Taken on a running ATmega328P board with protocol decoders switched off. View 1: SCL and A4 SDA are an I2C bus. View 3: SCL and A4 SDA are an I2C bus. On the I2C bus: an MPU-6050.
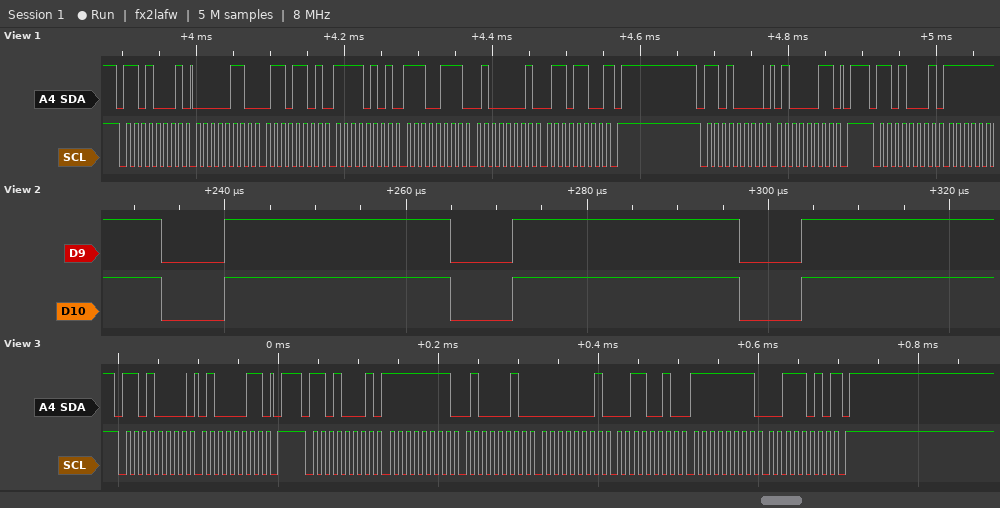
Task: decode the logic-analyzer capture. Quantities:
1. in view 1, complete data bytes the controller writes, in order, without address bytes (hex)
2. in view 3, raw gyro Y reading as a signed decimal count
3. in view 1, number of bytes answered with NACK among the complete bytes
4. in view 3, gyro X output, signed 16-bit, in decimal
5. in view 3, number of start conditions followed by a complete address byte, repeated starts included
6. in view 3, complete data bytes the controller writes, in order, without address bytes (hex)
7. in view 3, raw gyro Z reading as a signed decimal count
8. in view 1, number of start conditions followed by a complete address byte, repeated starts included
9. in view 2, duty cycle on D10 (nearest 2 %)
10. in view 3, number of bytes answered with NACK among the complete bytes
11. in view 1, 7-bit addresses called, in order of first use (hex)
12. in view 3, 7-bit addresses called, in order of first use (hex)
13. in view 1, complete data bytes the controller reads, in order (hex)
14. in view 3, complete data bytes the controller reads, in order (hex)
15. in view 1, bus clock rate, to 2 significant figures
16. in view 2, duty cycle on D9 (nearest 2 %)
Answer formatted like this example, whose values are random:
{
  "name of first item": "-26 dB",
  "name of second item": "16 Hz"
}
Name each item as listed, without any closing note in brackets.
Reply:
{
  "in view 1, complete data bytes the controller writes, in order, without address bytes": "43",
  "in view 3, raw gyro Y reading as a signed decimal count": "306",
  "in view 1, number of bytes answered with NACK among the complete bytes": "1",
  "in view 3, gyro X output, signed 16-bit, in decimal": "-190",
  "in view 3, number of start conditions followed by a complete address byte, repeated starts included": "2",
  "in view 3, complete data bytes the controller writes, in order, without address bytes": "43",
  "in view 3, raw gyro Z reading as a signed decimal count": "-198",
  "in view 1, number of start conditions followed by a complete address byte, repeated starts included": "3",
  "in view 2, duty cycle on D10": "78 %",
  "in view 3, number of bytes answered with NACK among the complete bytes": "1",
  "in view 1, 7-bit addresses called, in order of first use": "0x68",
  "in view 3, 7-bit addresses called, in order of first use": "0x68",
  "in view 1, complete data bytes the controller reads, in order": "06 6D F5 E7 41 6C",
  "in view 3, complete data bytes the controller reads, in order": "FF 42 01 32 FF 3A",
  "in view 1, bus clock rate, to 2 significant figures": "100 kHz",
  "in view 2, duty cycle on D9": "78 %"
}
